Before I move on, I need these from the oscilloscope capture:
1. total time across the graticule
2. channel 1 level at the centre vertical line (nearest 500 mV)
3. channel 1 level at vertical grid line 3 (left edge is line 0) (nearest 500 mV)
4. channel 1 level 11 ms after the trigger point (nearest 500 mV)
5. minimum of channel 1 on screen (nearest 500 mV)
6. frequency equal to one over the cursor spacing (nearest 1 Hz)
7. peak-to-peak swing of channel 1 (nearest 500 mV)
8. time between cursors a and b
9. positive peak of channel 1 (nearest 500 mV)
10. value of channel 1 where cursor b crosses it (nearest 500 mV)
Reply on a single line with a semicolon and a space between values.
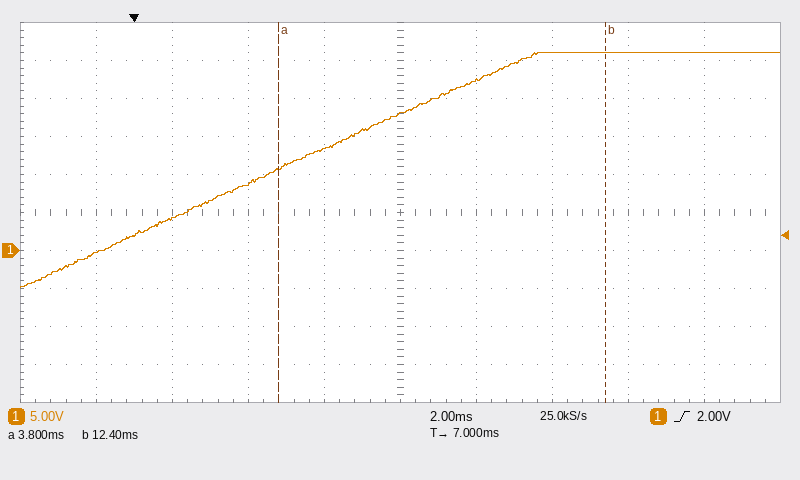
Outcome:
20 ms; 18.0 V; 9.0 V; 26.0 V; -5.0 V; 116 Hz; 31.0 V; 8.6 ms; 26.0 V; 26.0 V
